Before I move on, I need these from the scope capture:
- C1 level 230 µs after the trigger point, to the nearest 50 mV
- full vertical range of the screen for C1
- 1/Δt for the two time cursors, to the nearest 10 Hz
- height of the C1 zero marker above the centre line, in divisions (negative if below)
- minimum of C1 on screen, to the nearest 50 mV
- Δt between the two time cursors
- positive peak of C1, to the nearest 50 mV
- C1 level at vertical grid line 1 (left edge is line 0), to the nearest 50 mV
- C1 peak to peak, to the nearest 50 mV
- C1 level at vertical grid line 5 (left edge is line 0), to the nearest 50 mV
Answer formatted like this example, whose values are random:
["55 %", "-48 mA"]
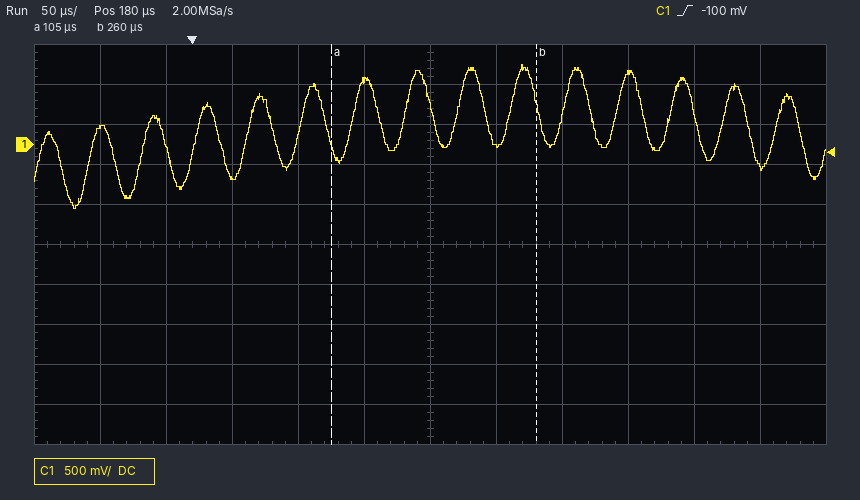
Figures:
["0 mV", "5 V", "6.45 kHz", "+2.5 div", "-800 mV", "155 µs", "1.00 V", "200 mV", "1.80 V", "800 mV"]
